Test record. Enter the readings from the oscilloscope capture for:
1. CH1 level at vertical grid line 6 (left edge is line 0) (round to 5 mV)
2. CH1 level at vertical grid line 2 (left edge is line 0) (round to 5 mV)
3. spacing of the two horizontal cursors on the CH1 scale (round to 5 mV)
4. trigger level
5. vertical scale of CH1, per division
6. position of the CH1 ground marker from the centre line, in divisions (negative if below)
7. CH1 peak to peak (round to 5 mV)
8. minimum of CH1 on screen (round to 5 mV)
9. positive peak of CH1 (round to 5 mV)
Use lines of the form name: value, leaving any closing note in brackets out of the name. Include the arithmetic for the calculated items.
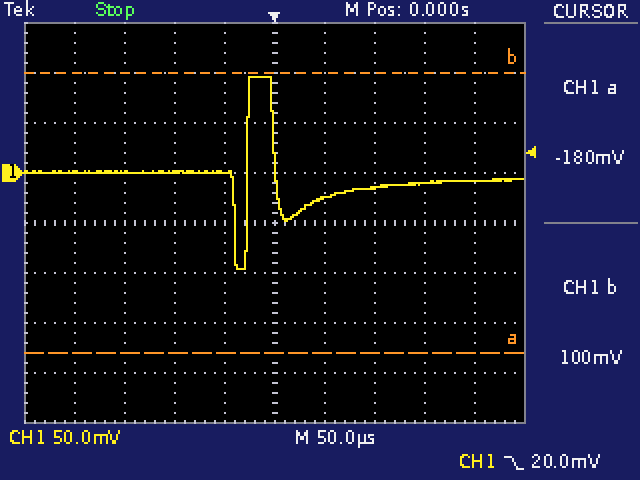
CH1 level at vertical grid line 6 (left edge is line 0): -25 mV
CH1 level at vertical grid line 2 (left edge is line 0): 0 mV
spacing of the two horizontal cursors on the CH1 scale: 280 mV
trigger level: 20.0 mV
vertical scale of CH1, per division: 50 mV
position of the CH1 ground marker from the centre line, in divisions: +1.0 div
CH1 peak to peak: 95 mV − (-95 mV) = 190 mV
minimum of CH1 on screen: -95 mV
positive peak of CH1: 95 mV
